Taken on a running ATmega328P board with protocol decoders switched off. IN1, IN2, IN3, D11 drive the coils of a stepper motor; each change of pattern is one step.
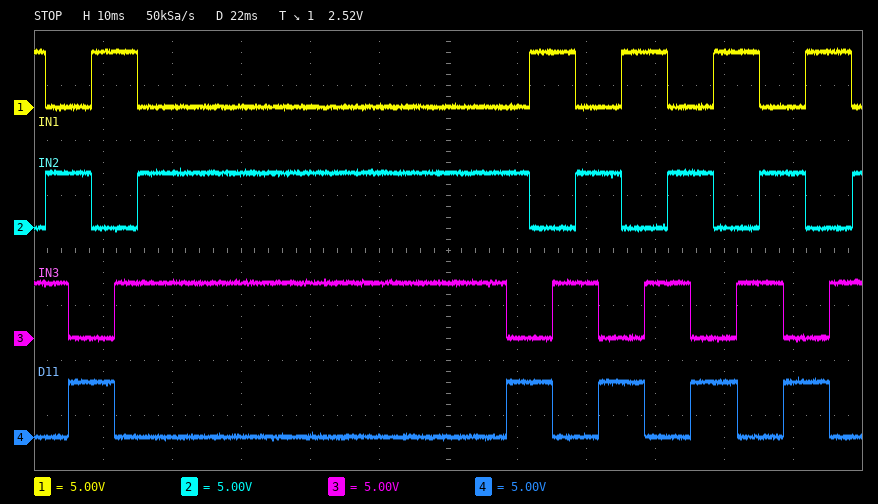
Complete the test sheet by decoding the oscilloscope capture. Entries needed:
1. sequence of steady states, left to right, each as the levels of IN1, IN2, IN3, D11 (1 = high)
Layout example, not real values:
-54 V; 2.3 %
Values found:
1010 0110 0101 1001 1010 0110 0101 1001 1010 0110 0101 1001 1010 0110 0101 1001 1010 0110 0101 1001 1010 0110
